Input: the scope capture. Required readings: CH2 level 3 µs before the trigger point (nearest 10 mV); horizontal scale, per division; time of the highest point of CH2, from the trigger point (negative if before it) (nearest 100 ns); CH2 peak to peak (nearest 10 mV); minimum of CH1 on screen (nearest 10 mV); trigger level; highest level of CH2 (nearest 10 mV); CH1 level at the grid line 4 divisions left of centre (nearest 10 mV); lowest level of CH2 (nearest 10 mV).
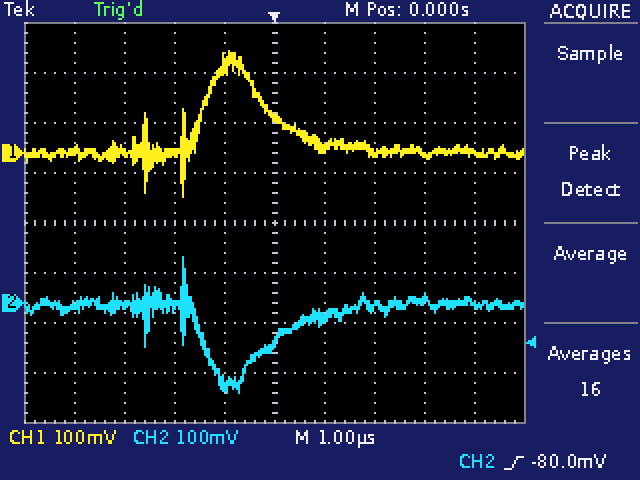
0 mV
1 µs
-1.8 µs
270 mV
-90 mV
-80.0 mV
90 mV
10 mV
-180 mV
